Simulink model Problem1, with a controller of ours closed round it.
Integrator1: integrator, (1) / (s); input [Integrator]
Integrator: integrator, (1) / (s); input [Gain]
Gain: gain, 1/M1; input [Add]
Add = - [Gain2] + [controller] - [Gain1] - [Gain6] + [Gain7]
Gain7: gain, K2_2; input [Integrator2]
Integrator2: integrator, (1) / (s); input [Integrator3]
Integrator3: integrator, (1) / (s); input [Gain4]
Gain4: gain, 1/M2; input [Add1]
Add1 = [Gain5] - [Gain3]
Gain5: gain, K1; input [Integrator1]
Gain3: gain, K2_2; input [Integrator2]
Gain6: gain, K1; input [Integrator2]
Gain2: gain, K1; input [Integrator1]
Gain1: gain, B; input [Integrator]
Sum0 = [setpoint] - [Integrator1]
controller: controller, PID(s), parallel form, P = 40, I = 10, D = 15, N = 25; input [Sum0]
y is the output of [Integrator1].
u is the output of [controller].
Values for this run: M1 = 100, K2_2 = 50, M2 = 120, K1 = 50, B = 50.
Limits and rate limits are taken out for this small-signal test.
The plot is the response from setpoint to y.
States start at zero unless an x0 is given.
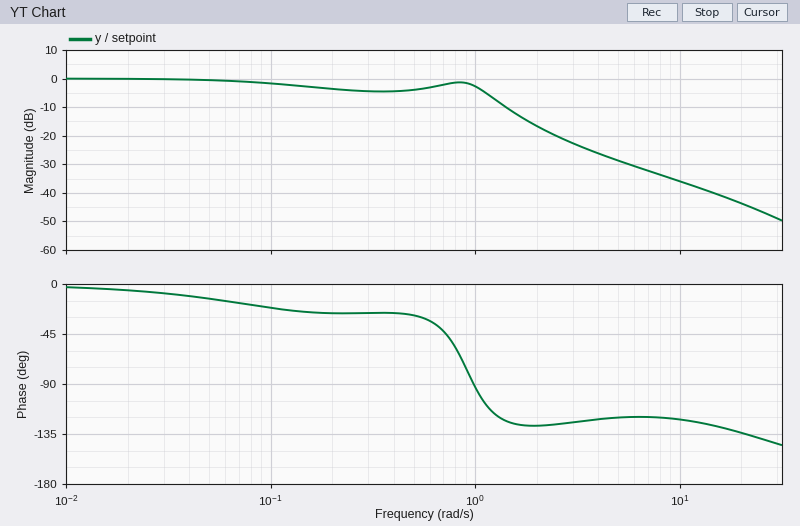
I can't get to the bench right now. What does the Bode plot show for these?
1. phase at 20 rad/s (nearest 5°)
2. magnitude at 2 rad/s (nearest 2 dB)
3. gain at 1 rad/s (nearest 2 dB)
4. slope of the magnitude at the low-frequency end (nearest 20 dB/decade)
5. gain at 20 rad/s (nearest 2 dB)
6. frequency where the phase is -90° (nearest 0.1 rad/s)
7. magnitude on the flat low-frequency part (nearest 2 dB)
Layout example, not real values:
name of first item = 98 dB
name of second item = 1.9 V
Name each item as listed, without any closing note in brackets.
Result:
phase at 20 rad/s = -135°
magnitude at 2 rad/s = -16 dB
gain at 1 rad/s = -2 dB
slope of the magnitude at the low-frequency end = 0 dB/decade
gain at 20 rad/s = -44 dB
frequency where the phase is -90° = 1.0 rad/s
magnitude on the flat low-frequency part = 0 dB
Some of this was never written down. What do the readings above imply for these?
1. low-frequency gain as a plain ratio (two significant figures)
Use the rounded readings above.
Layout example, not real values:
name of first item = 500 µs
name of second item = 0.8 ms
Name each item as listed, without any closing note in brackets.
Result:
low-frequency gain as a plain ratio = 1.0
